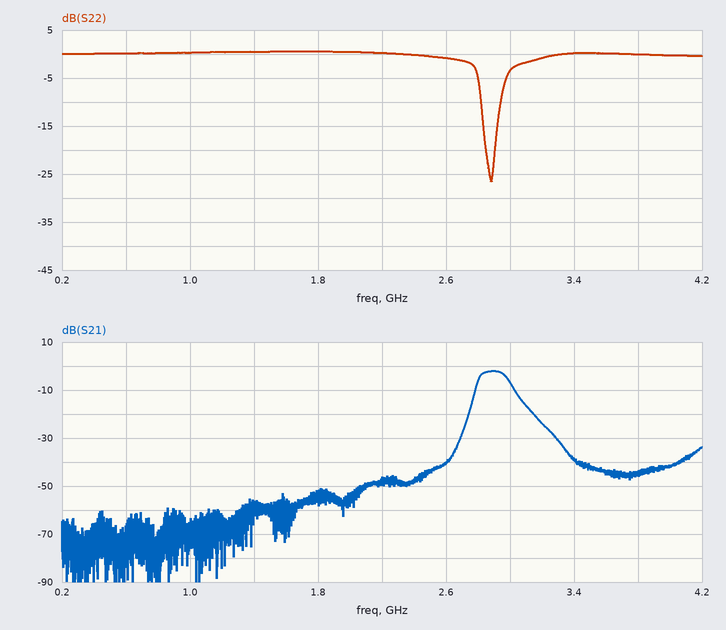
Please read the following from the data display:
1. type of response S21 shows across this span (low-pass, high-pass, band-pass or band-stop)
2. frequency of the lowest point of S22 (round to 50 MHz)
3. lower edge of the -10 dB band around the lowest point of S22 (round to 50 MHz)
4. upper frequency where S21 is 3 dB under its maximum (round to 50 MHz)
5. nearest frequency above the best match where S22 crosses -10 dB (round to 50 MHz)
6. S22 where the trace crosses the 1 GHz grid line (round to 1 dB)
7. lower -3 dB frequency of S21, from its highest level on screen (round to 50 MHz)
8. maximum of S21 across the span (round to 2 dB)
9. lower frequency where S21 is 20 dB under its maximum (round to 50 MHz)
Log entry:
band-pass
2.90 GHz
2.80 GHz
3.00 GHz
2.95 GHz
0 dB
2.80 GHz
-2 dB
2.75 GHz
